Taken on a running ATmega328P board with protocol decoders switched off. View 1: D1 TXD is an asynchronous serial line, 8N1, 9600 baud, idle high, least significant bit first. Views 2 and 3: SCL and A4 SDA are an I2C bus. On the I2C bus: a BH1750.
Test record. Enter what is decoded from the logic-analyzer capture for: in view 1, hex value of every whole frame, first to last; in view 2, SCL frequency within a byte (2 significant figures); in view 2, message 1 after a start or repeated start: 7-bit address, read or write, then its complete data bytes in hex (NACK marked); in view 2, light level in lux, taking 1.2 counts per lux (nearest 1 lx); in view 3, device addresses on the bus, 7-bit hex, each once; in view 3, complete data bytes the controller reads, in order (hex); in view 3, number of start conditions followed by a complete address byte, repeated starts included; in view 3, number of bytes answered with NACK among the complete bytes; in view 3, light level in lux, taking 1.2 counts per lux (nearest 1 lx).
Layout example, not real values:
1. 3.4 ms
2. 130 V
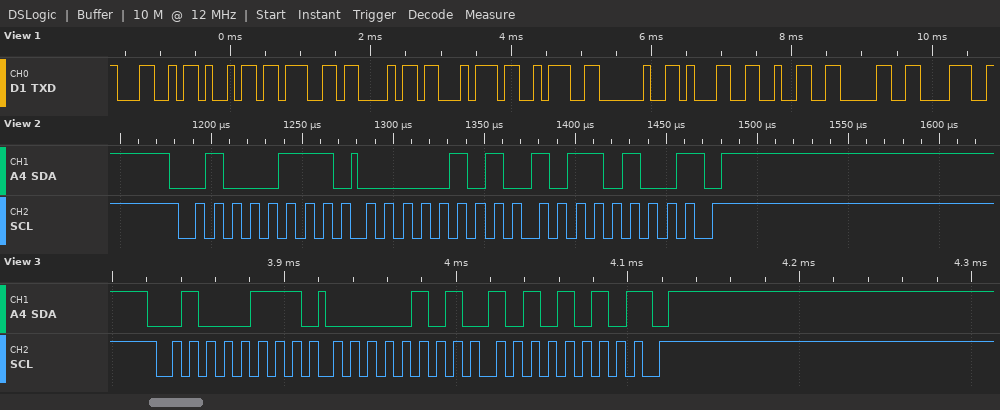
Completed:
1. 4C 69 67 68 74 3A 20 31 32 30 38
2. 100 kHz
3. 0x23 read: 05 B4 NACK
4. 1217 lx
5. 0x23
6. 05 AA
7. 1
8. 1
9. 1208 lx
